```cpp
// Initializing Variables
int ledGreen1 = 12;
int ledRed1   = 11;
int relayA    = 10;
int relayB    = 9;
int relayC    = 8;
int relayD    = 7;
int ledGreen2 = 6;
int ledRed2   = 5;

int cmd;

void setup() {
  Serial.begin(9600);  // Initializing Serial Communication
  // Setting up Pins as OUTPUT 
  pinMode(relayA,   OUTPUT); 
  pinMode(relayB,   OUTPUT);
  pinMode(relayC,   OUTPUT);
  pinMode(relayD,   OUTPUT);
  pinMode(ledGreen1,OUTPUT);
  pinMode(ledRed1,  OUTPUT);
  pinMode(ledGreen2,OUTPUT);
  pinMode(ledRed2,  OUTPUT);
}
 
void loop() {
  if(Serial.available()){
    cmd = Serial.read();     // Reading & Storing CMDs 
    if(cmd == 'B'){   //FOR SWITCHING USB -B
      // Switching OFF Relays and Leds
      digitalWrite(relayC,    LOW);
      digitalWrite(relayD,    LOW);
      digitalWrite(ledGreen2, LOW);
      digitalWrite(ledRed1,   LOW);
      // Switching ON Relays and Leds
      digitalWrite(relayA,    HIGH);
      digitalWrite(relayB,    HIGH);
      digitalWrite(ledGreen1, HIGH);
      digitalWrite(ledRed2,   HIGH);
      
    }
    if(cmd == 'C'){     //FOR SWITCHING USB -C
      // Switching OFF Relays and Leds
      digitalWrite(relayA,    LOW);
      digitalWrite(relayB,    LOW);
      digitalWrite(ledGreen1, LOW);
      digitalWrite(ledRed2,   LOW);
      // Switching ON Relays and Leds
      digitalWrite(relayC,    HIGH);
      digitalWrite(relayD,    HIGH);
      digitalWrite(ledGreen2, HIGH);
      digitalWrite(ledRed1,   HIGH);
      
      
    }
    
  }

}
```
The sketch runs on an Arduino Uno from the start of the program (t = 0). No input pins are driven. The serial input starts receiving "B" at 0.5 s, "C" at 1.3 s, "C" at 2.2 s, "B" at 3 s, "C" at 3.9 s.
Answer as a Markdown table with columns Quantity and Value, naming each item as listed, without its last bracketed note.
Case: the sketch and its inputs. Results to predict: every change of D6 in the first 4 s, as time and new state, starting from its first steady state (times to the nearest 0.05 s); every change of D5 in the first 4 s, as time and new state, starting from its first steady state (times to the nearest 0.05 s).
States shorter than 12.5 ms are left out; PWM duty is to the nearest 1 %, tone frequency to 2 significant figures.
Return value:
| Quantity | Value |
|---|---|
| every change of D6 in the first 4 s, as time and new state, starting from its first steady state | 0 s low; 1.3 s high; 3 s low; 3.9 s high |
| every change of D5 in the first 4 s, as time and new state, starting from its first steady state | 0 s low; 0.5 s high; 1.3 s low; 3 s high; 3.9 s low |
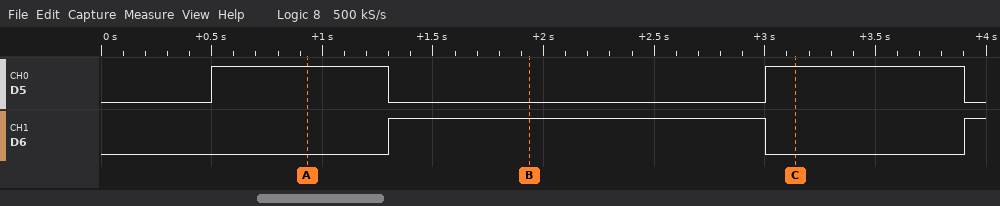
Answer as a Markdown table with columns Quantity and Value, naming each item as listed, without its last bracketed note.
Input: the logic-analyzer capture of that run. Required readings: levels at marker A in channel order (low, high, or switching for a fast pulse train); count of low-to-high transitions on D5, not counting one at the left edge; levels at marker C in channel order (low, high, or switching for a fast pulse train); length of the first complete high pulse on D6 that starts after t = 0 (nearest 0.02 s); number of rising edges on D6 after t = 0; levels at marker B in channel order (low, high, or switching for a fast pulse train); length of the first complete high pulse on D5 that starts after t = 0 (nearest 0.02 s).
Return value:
| Quantity | Value |
|---|---|
| levels at marker A in channel order | D5 high, D6 low |
| count of low-to-high transitions on D5, not counting one at the left edge | 2 |
| levels at marker C in channel order | D5 high, D6 low |
| length of the first complete high pulse on D6 that starts after t = 0 | 1.70 s |
| number of rising edges on D6 after t = 0 | 2 |
| levels at marker B in channel order | D5 low, D6 high |
| length of the first complete high pulse on D5 that starts after t = 0 | 0.80 s |
